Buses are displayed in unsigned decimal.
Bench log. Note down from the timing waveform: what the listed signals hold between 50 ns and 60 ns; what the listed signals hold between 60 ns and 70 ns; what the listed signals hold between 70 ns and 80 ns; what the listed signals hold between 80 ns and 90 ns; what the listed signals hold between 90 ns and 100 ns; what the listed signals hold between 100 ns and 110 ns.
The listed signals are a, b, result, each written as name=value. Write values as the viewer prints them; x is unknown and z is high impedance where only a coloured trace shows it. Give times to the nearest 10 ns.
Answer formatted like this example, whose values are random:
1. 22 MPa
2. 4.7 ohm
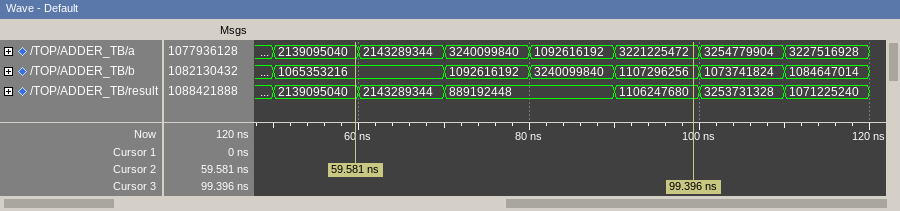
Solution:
1. a=2139095040, b=1065353216, result=2139095040
2. a=2143289344, b=1065353216, result=2143289344
3. a=3240099840, b=1092616192, result=889192448
4. a=1092616192, b=3240099840, result=889192448
5. a=3221225472, b=1107296256, result=1106247680
6. a=3254779904, b=1073741824, result=3253731328
